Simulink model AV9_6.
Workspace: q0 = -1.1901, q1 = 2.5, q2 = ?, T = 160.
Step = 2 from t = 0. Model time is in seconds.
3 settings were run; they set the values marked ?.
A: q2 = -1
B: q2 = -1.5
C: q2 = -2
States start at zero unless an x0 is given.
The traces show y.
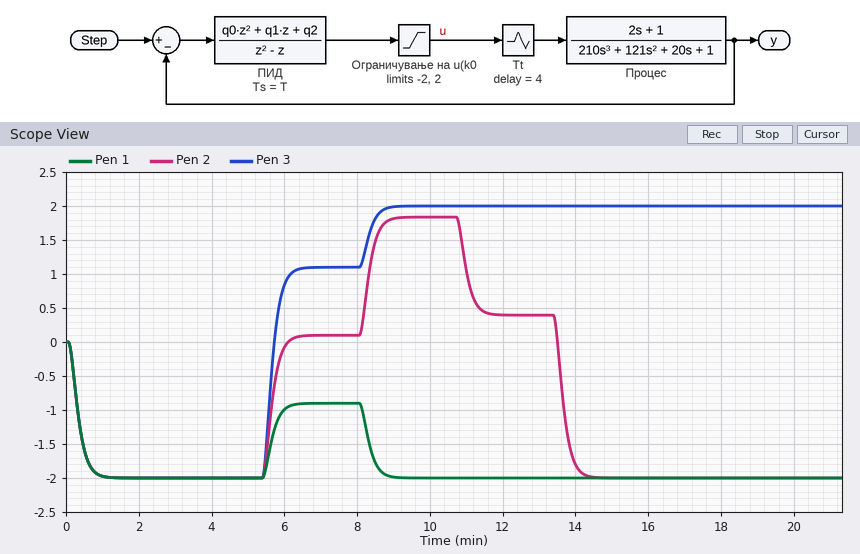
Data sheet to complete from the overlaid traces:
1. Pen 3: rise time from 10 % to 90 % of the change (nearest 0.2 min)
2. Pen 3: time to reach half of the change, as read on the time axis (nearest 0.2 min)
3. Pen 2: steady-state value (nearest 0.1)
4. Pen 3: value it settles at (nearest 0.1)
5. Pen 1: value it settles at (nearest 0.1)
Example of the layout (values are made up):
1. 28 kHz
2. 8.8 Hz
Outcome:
1. 2.8 min
2. 6.2 min
3. -2.0
4. 2.0
5. -2.0
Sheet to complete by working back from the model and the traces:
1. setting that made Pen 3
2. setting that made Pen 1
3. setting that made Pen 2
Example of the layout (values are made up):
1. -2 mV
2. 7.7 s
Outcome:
1. A
2. C
3. B
